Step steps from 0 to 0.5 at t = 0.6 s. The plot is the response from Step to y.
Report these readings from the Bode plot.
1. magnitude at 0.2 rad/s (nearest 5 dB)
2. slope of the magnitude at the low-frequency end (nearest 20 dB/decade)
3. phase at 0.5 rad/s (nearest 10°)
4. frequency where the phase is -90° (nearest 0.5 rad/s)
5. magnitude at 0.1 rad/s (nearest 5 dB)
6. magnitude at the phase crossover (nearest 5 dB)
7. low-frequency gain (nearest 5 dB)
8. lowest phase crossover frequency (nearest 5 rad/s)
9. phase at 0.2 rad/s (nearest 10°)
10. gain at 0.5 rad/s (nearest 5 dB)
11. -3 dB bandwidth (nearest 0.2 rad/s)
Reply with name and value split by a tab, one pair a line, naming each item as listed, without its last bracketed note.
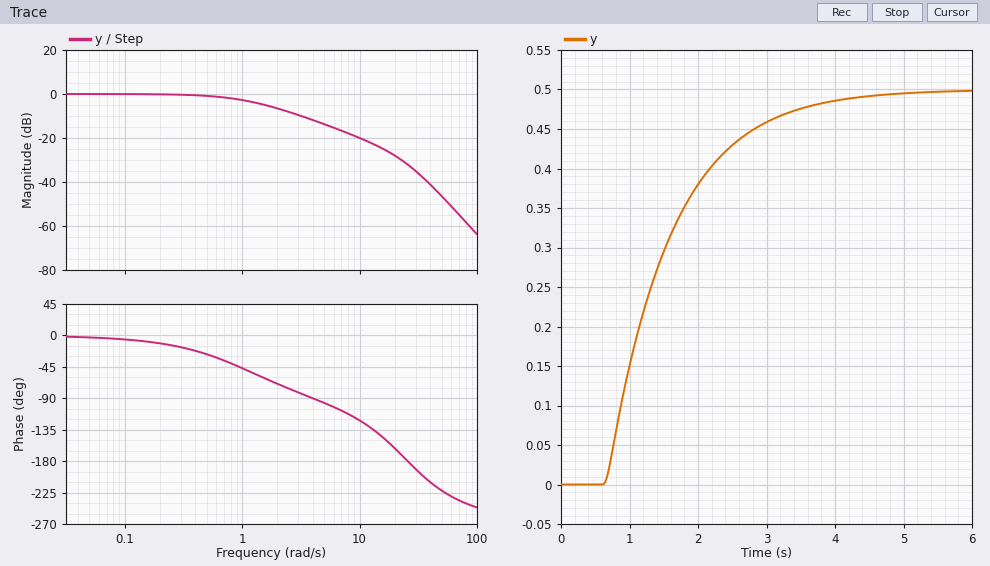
magnitude at 0.2 rad/s	0 dB
slope of the magnitude at the low-frequency end	0 dB/decade
phase at 0.5 rad/s	-30°
frequency where the phase is -90°	4.0 rad/s
magnitude at 0.1 rad/s	0 dB
magnitude at the phase crossover	-30 dB
low-frequency gain	0 dB
lowest phase crossover frequency	25 rad/s
phase at 0.2 rad/s	-10°
gain at 0.5 rad/s	0 dB
-3 dB bandwidth	1.0 rad/s
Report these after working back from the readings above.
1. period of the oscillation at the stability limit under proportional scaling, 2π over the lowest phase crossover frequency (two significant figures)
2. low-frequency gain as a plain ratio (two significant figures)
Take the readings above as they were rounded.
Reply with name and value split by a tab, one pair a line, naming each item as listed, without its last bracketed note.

period of the oscillation at the stability limit under proportional scaling, 2π over the lowest phase crossover frequency	0.25 s
low-frequency gain as a plain ratio	1.0
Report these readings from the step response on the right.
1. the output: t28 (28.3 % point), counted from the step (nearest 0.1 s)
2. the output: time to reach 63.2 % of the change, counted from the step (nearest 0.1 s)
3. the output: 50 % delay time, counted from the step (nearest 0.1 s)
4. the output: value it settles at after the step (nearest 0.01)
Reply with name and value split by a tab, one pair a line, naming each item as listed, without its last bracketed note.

the output: t28 (28.3 % point), counted from the step	0.4 s
the output: time to reach 63.2 % of the change, counted from the step	1.0 s
the output: 50 % delay time, counted from the step	0.7 s
the output: value it settles at after the step	0.50
